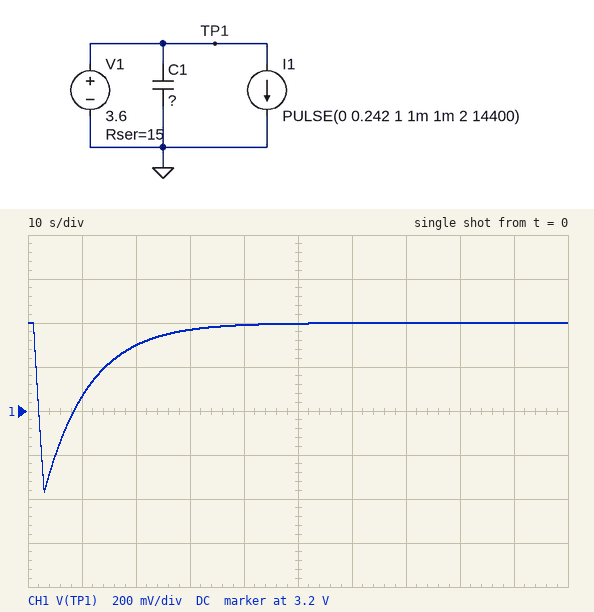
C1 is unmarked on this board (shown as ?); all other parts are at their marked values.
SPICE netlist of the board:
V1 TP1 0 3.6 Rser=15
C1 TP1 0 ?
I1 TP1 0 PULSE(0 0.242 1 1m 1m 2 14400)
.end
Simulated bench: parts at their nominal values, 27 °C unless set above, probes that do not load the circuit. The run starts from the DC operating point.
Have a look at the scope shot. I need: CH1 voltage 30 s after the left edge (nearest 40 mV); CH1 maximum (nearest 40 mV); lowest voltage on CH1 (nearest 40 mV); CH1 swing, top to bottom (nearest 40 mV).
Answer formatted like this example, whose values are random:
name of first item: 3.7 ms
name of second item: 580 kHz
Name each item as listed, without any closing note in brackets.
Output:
CH1 voltage 30 s after the left edge: 3.56 V
CH1 maximum: 3.60 V
lowest voltage on CH1: 2.84 V
CH1 swing, top to bottom: 760 mV
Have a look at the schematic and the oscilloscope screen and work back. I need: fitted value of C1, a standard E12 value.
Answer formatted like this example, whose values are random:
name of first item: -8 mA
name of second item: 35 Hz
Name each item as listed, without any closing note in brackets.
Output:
fitted value of C1, a standard E12 value: 560 mF
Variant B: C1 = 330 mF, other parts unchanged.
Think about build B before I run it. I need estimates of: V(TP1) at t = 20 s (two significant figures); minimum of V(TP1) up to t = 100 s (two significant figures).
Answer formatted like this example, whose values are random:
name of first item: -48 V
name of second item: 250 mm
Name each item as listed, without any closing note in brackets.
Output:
V(TP1) at t = 20 s: 3.6 V
minimum of V(TP1) up to t = 100 s: 2.4 V
